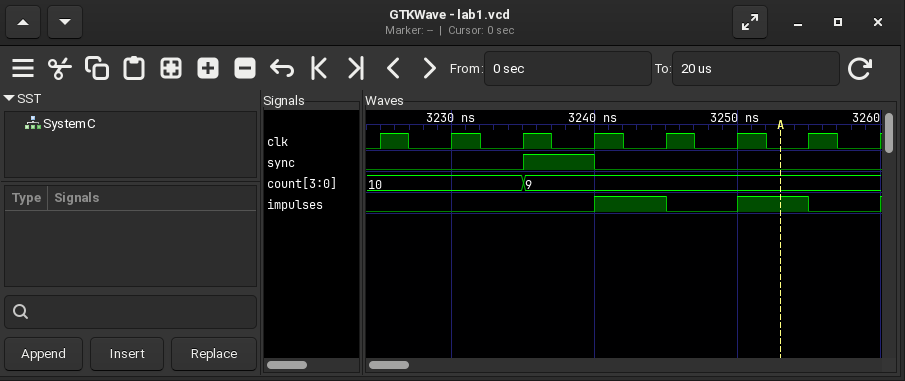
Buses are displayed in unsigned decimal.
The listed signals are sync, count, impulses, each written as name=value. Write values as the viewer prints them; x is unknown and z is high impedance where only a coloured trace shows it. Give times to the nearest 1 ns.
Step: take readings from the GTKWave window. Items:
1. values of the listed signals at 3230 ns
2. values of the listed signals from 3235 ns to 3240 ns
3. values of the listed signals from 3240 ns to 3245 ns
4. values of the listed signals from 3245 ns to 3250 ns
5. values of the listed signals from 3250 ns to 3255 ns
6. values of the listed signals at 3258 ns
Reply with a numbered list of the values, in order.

1. sync=0, count=10, impulses=0
2. sync=1, count=9, impulses=0
3. sync=0, count=9, impulses=1
4. sync=0, count=9, impulses=0
5. sync=0, count=9, impulses=1
6. sync=0, count=9, impulses=0
